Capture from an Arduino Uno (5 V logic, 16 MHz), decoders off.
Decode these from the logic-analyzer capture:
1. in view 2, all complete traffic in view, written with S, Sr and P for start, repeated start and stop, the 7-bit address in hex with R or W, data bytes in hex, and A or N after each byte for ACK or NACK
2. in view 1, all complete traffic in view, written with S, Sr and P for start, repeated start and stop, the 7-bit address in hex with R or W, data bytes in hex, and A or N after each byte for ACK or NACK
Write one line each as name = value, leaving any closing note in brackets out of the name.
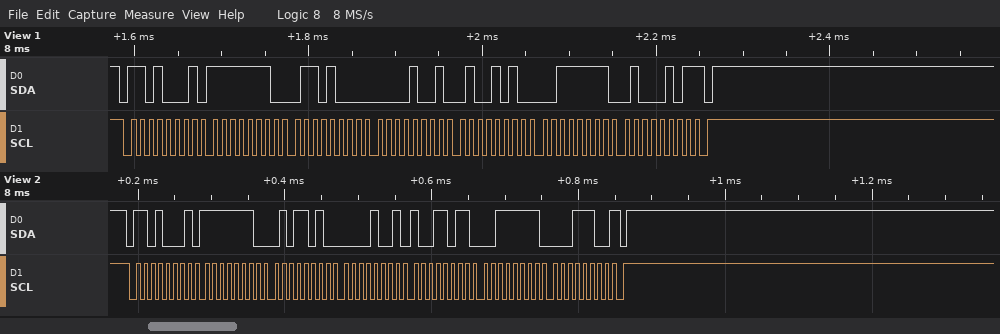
in view 2, all complete traffic in view, written with S, Sr and P for start, repeated start and stop, the 7-bit address in hex with R or W, data bytes in hex, and A or N after each byte for ACK or NACK = S 68R A FE A 5A A 09 A 9B A 3F A 1C N P
in view 1, all complete traffic in view, written with S, Sr and P for start, repeated start and stop, the 7-bit address in hex with R or W, data bytes in hex, and A or N after each byte for ACK or NACK = S 68R A FE A 68 A 09 A 4A A 3F A 45 N P
